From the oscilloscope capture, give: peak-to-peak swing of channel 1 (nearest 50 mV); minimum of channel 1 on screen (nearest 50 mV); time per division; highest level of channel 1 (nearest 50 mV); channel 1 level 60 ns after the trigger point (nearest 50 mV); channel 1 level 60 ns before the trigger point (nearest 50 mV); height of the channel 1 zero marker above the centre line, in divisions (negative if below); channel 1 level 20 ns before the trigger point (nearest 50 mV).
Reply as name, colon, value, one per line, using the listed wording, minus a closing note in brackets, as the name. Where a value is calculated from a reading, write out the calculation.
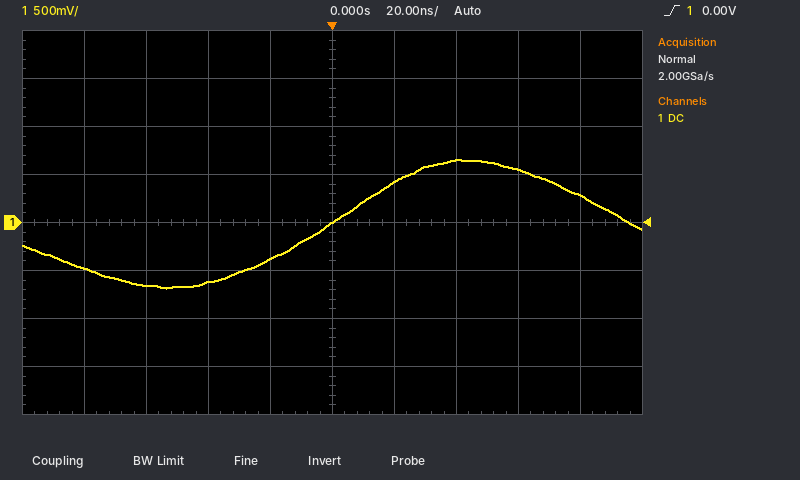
peak-to-peak swing of channel 1: 650 mV − (-700 mV) = 1.35 V
minimum of channel 1 on screen: -700 mV
time per division: 20 ns
highest level of channel 1: 650 mV
channel 1 level 60 ns after the trigger point: 550 mV
channel 1 level 60 ns before the trigger point: -650 mV
height of the channel 1 zero marker above the centre line, in divisions: 0.0 div
channel 1 level 20 ns before the trigger point: -400 mV
